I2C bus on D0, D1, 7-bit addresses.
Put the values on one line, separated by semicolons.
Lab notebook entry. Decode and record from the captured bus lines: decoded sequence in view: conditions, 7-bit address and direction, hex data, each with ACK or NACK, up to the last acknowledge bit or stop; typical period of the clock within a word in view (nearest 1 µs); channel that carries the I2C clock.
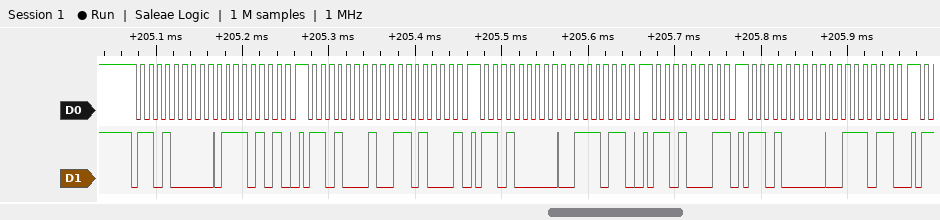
start, address 68 write ACK, 75 ACK, stop, start, address 68 read ACK, 68 NACK, stop, start, address 68 write ACK, 3B ACK, stop, start, address 68 read NACK, stop, start, address 68 write ACK, 3B ACK, stop; 10 µs; D0
